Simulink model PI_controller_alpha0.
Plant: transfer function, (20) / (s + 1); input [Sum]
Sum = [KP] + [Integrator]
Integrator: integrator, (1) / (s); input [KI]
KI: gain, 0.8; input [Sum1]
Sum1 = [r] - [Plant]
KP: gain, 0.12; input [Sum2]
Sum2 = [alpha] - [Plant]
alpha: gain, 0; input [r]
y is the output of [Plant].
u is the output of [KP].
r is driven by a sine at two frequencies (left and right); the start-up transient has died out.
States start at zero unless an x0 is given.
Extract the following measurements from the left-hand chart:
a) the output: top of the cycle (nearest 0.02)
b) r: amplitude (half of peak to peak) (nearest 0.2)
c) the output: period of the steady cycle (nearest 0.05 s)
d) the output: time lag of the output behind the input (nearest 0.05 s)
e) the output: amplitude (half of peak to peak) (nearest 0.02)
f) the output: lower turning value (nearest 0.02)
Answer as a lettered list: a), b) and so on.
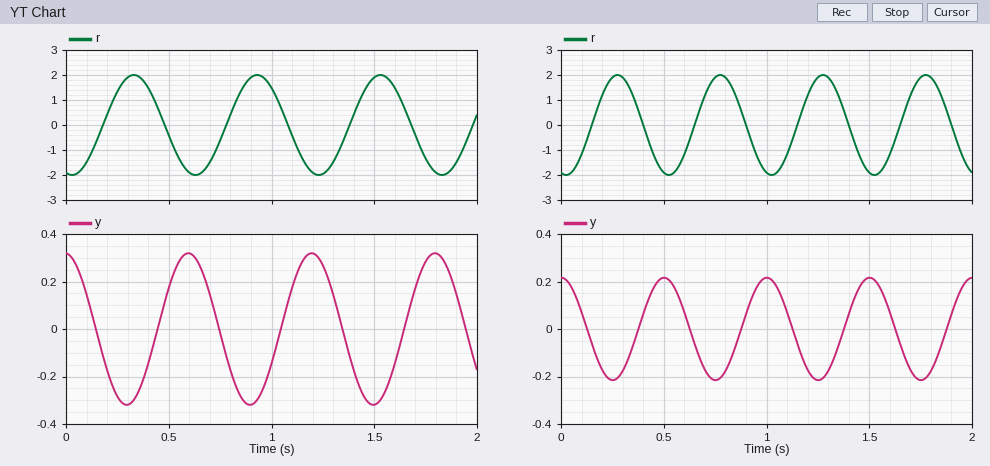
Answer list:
a) 0.32
b) 2.0
c) 0.60 s
d) 0.25 s
e) 0.32
f) -0.32
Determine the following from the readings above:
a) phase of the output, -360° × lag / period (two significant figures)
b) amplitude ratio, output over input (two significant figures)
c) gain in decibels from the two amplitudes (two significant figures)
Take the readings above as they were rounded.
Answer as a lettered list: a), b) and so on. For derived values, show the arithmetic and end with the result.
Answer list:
a) -360 × 0.25 / 0.6 = -150°
b) 0.32 / 2 = 0.16
c) 20 log10(0.32 / 2) = -16 dB
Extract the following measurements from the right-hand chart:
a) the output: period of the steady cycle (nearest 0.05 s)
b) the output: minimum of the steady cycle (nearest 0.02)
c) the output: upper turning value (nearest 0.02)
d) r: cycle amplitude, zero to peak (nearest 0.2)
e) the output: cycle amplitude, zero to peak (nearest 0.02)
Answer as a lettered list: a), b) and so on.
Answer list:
a) 0.50 s
b) -0.22
c) 0.22
d) 2.0
e) 0.22
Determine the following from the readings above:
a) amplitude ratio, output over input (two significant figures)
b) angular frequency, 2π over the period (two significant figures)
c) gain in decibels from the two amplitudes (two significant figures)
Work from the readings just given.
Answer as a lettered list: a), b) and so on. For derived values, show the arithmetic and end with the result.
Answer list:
a) 0.22 / 2 = 0.11
b) 2π / 0.5 = 13 rad/s
c) 20 log10(0.22 / 2) = -19 dB
